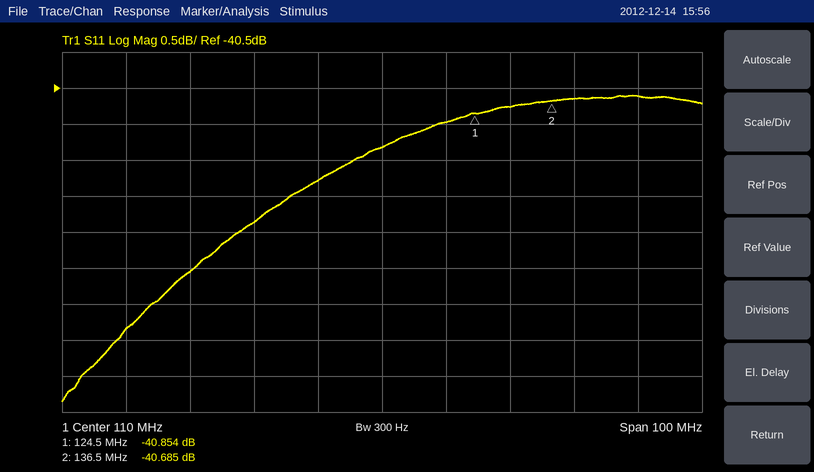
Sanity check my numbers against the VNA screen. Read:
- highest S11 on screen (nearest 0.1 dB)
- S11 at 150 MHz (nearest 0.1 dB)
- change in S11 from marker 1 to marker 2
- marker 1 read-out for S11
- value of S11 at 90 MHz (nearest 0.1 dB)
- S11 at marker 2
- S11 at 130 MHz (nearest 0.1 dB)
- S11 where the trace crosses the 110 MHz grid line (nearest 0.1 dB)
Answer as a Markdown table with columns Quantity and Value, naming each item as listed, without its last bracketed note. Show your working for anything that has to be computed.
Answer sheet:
| Quantity | Value |
|---|---|
| highest S11 on screen | -40.6 dB |
| S11 at 150 MHz | -40.6 dB |
| change in S11 from marker 1 to marker 2 | -40.685 − (-40.854) = 0.169 dB |
| marker 1 read-out for S11 | -40.854 dB |
| value of S11 at 90 MHz | -42.4 dB |
| S11 at marker 2 | -40.685 dB |
| S11 at 130 MHz | -40.8 dB |
| S11 where the trace crosses the 110 MHz grid line | -41.3 dB |
